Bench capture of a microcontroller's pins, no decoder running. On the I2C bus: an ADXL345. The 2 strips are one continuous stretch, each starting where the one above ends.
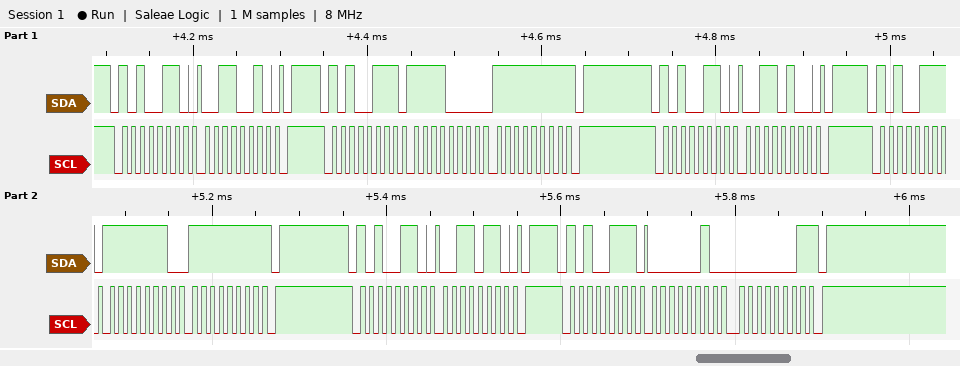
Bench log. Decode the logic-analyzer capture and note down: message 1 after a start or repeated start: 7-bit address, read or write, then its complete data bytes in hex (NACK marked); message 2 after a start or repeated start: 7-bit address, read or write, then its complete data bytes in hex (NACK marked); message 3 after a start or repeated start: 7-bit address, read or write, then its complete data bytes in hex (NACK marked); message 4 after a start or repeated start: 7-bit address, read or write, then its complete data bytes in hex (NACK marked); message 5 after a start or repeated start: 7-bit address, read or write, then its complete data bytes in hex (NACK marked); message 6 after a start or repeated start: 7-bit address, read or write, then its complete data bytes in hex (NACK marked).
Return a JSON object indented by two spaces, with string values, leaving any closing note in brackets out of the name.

{
  "message 1 after a start or repeated start: 7-bit address, read or write, then its complete data bytes in hex": "0x53 write: 32",
  "message 2 after a start or repeated start: 7-bit address, read or write, then its complete data bytes in hex": "0x53 read: F0 FF NACK",
  "message 3 after a start or repeated start: 7-bit address, read or write, then its complete data bytes in hex": "0x53 write: 34",
  "message 4 after a start or repeated start: 7-bit address, read or write, then its complete data bytes in hex": "0x53 read: FE FF NACK",
  "message 5 after a start or repeated start: 7-bit address, read or write, then its complete data bytes in hex": "0x53 write: 36",
  "message 6 after a start or repeated start: 7-bit address, read or write, then its complete data bytes in hex": "0x53 read: 02 01 NACK"
}
